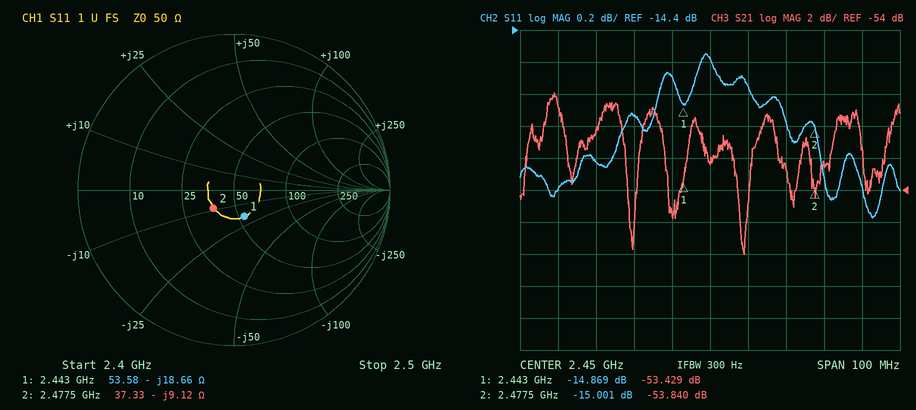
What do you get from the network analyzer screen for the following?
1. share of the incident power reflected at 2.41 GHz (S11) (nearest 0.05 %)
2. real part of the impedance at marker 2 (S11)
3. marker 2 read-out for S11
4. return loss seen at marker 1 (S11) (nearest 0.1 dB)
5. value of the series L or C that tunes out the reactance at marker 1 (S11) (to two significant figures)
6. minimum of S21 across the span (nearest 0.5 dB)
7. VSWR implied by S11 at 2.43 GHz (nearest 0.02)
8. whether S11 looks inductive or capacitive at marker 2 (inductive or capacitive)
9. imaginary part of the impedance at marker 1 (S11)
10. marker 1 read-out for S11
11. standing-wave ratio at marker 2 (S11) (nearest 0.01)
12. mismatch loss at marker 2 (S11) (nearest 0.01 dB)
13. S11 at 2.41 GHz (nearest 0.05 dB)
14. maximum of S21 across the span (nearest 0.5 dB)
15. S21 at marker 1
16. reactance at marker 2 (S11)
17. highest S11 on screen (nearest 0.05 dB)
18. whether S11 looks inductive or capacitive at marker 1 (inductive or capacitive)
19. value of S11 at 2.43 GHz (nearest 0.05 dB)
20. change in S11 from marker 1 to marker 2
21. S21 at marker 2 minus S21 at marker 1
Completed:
2.90 %
37.33 Ω
-15.001 dB
14.9 dB
1.2 nH
-58.0 dB
1.44
capacitive
-18.66 Ω
-14.869 dB
1.43
0.14 dB
-15.40 dB
-48.0 dB
-53.429 dB
-9.12 Ω
-14.55 dB
capacitive
-14.95 dB
-0.132 dB
-0.411 dB
